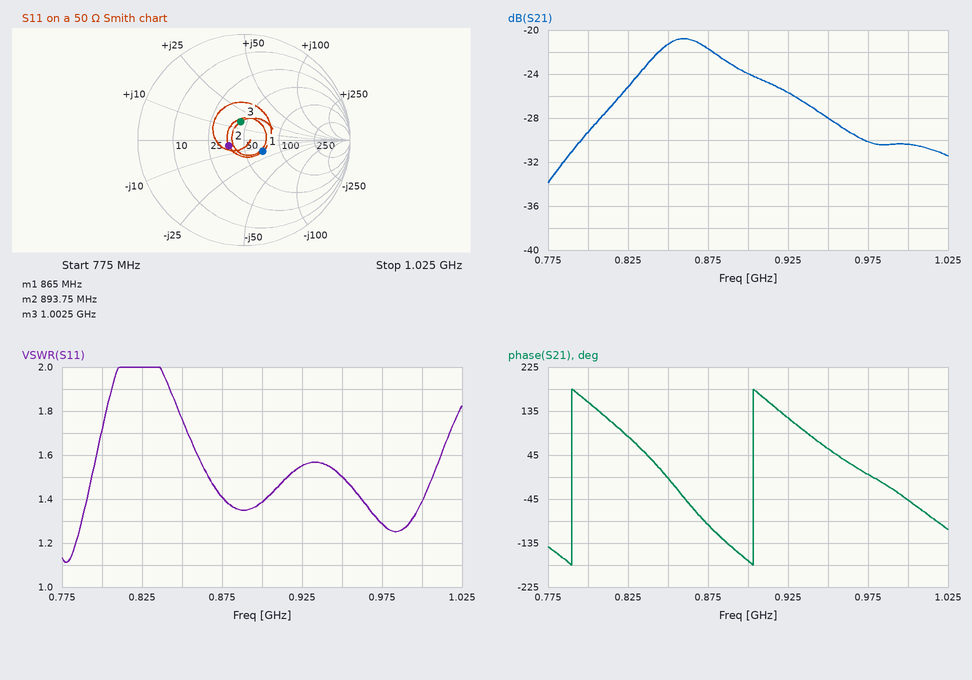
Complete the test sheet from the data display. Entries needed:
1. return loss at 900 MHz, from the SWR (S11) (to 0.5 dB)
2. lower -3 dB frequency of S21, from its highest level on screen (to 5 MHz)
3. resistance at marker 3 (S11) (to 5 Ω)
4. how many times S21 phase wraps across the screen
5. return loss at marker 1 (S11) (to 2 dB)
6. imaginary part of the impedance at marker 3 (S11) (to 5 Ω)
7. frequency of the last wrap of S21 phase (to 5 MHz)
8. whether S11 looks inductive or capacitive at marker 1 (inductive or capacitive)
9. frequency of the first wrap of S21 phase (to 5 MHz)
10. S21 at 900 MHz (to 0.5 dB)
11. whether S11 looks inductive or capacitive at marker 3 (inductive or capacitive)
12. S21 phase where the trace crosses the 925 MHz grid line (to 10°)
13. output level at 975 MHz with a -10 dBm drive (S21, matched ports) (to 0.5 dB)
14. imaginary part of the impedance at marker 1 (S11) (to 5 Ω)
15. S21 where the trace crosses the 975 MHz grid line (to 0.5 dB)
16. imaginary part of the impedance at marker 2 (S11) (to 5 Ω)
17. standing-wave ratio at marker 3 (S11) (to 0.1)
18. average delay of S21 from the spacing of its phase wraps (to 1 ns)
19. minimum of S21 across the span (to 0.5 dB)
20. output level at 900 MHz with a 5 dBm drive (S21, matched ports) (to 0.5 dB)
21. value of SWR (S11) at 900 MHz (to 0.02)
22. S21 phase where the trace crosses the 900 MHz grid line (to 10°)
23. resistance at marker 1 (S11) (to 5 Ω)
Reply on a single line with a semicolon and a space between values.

16.0 dB; 835 MHz; 45 Ω; 2; 14 dB; +15 Ω; 905 MHz; capacitive; 790 MHz; -24.0 dB; inductive; 120°; -40.0 dBm; -15 Ω; -30.0 dB; -5 Ω; 1.4; 9 ns; -34.0 dB; -19.0 dBm; 1.38; -170°; 70 Ω
